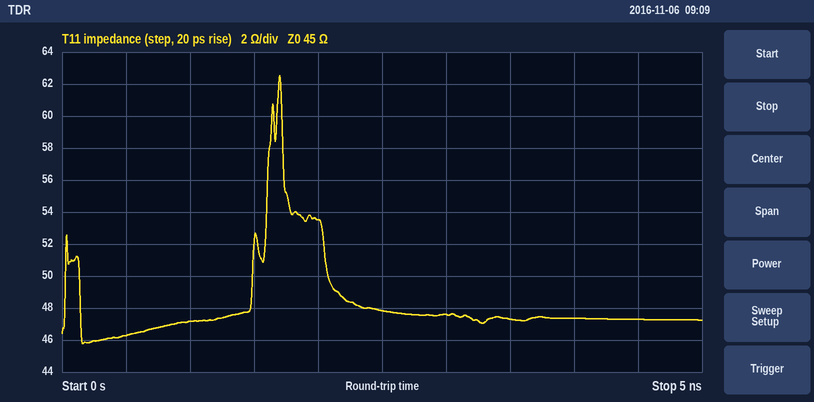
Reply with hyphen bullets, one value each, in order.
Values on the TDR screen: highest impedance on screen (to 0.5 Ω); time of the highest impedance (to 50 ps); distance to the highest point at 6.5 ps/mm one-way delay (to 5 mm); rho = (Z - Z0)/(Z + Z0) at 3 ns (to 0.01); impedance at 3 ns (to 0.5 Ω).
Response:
- 62.5 Ω
- 1.70 ns
- 130 mm
- +0.03
- 47.5 Ω
